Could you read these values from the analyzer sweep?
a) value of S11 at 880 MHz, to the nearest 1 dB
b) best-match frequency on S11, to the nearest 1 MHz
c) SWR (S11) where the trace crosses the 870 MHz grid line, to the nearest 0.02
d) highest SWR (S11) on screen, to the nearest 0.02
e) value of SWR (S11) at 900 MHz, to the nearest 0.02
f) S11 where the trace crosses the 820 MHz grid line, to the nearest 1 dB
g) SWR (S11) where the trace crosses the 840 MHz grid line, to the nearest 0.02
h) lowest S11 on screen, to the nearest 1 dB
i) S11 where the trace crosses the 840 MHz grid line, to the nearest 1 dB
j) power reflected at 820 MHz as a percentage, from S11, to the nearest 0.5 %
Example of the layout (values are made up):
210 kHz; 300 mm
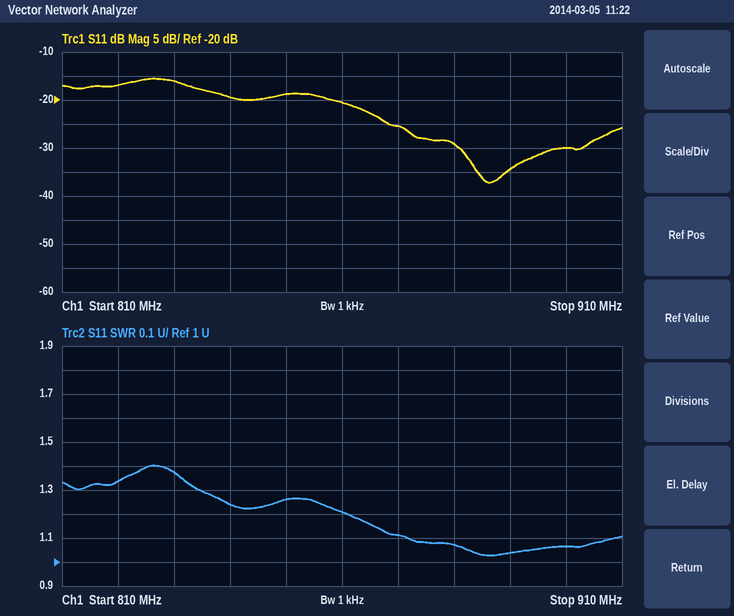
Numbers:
-29 dB; 886 MHz; 1.12; 1.40; 1.06; -17 dB; 1.24; -37 dB; -19 dB; 2.0 %
